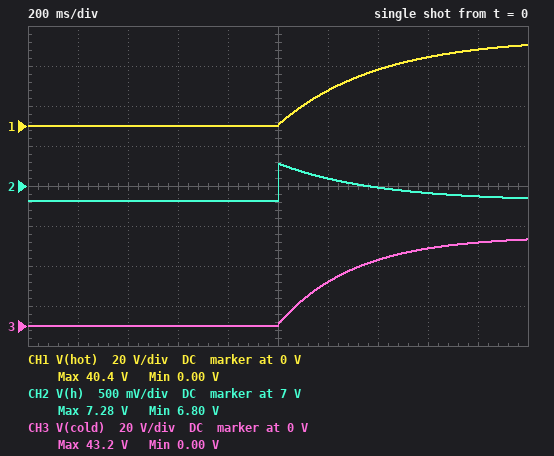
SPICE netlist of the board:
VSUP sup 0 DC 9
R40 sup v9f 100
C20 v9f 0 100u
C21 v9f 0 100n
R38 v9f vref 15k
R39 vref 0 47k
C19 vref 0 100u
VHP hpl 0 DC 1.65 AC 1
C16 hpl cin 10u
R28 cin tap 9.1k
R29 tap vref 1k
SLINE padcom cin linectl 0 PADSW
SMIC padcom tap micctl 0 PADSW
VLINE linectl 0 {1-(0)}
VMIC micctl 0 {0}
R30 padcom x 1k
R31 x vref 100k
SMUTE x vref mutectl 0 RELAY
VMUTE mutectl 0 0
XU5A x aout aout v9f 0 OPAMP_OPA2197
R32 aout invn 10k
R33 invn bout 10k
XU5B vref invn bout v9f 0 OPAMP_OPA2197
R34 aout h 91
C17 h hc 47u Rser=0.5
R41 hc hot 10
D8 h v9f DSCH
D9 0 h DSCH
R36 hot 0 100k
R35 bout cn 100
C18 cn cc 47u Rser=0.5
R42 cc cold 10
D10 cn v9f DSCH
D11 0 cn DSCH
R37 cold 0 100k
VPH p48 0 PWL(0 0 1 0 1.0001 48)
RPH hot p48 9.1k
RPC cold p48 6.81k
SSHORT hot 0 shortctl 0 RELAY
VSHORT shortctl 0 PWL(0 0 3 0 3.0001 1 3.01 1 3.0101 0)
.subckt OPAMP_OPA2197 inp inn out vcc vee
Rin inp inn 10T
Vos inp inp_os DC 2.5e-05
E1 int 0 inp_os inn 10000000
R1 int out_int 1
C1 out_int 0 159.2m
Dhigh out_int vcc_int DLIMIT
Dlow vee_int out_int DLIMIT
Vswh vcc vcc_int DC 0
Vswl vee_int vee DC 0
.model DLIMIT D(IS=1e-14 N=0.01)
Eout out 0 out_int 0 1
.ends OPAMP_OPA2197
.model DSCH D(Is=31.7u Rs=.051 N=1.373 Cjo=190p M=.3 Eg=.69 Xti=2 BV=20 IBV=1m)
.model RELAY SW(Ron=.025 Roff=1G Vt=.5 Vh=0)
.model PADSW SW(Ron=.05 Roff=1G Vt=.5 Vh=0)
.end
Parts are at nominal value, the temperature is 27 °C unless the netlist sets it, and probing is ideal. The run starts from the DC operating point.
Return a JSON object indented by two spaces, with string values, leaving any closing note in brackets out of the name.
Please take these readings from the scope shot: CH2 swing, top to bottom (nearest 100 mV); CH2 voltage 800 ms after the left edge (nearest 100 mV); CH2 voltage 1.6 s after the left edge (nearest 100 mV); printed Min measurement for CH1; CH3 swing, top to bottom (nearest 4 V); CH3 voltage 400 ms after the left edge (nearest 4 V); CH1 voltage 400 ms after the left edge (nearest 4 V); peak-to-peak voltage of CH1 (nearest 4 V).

{
  "CH2 swing, top to bottom": "500 mV",
  "CH2 voltage 800 ms after the left edge": "6.8 V",
  "CH2 voltage 1.6 s after the left edge": "6.9 V",
  "printed Min measurement for CH1": "0.00 V",
  "CH3 swing, top to bottom": "44 V",
  "CH3 voltage 400 ms after the left edge": "0 V",
  "CH1 voltage 400 ms after the left edge": "0 V",
  "peak-to-peak voltage of CH1": "40 V"
}
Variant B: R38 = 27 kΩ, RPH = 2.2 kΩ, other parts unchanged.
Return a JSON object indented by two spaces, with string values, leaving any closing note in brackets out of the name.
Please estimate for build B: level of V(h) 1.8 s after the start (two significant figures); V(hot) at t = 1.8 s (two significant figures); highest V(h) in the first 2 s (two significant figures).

{
  "level of V(h) 1.8 s after the start": "5.7 V",
  "V(hot) at t = 1.8 s": "47 V",
  "highest V(h) in the first 2 s": "7.6 V"
}
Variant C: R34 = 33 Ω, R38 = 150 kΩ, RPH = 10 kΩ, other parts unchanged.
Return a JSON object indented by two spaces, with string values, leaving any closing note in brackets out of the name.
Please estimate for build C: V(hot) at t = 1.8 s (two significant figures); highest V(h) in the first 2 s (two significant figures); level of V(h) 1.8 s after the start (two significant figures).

{
  "V(hot) at t = 1.8 s": "37 V",
  "highest V(h) in the first 2 s": "2.3 V",
  "level of V(h) 1.8 s after the start": "2.2 V"
}
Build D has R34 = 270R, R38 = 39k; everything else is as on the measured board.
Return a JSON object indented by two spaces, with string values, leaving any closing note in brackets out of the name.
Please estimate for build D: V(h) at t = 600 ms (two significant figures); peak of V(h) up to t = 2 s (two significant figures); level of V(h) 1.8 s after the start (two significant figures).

{
  "V(h) at t = 600 ms": "4.9 V",
  "peak of V(h) up to t = 2 s": "6.3 V",
  "level of V(h) 1.8 s after the start": "5.1 V"
}
